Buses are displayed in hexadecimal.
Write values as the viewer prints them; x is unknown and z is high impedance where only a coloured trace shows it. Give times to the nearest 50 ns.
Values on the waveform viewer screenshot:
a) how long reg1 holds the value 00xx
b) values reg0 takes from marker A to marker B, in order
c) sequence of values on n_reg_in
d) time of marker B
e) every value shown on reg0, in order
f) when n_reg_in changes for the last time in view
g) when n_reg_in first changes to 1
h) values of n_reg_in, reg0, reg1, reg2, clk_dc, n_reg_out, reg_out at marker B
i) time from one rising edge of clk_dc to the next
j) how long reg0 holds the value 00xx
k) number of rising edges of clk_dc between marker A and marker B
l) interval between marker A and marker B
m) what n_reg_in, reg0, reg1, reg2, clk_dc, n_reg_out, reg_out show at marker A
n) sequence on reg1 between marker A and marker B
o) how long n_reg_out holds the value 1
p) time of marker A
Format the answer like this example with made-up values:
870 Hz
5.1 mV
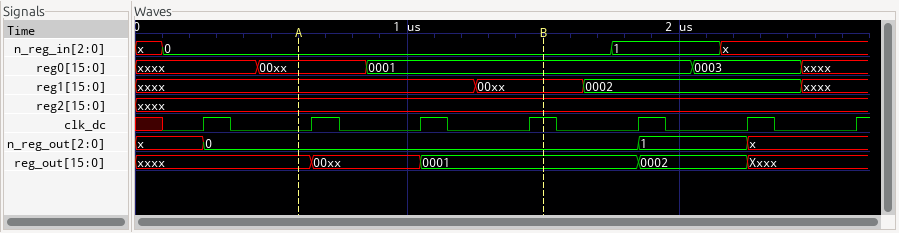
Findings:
400 ns
00xx, 0001
x, 0, 1, x
1500 ns
xxxx, 00xx, 0001, 0003, xxxx
2150 ns
1750 ns
n_reg_in=0, reg0=0001, reg1=00xx, reg2=xxxx, clk_dc=1, n_reg_out=0, reg_out=0001
400 ns
400 ns
3
900 ns
n_reg_in=0, reg0=00xx, reg1=xxxx, reg2=xxxx, clk_dc=0, n_reg_out=0, reg_out=xxxx
xxxx, 00xx
400 ns
600 ns
